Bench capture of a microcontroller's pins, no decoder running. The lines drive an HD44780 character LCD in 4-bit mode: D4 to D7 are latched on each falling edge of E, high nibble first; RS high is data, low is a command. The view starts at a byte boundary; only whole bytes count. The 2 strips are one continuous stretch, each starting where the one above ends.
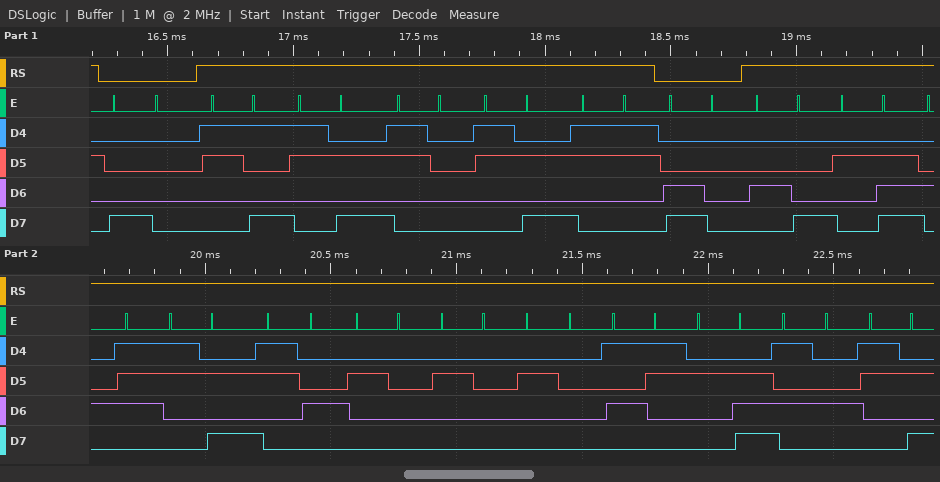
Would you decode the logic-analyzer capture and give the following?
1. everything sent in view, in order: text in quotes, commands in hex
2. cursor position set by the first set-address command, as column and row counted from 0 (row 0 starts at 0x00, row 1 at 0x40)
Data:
0x80 "9:0:3" 0xC0 "H.G:4   S.T:"
column 0, row 0
